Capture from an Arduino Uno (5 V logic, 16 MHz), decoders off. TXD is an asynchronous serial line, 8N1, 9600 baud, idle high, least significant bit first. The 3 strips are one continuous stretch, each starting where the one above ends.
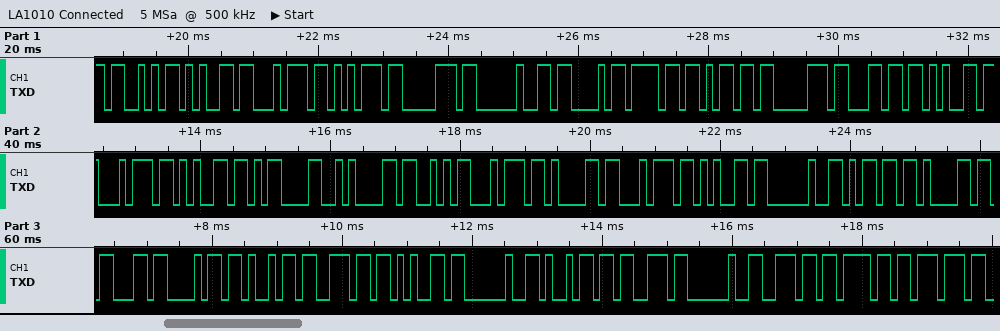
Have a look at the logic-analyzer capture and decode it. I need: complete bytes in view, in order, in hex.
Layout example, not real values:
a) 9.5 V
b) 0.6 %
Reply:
a) 53 65 74 75 70 20 43 6F 6D 70 6C 65 74 65 0D 0A 53 74 61 74 65 20 6D 61 63 68 69 6E 65 20 69 73 20 6E 6F 77
